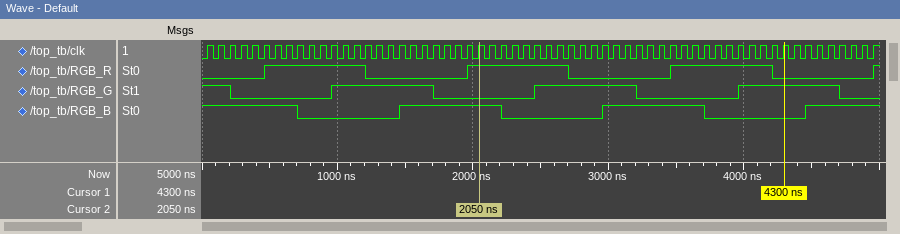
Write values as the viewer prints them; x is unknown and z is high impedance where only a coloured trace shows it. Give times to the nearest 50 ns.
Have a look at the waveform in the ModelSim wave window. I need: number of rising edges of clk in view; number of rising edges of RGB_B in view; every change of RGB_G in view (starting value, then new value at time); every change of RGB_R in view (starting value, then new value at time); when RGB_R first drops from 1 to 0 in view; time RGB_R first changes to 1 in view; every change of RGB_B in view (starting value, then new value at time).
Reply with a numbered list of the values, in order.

1. 60
2. 3
3. 1, 0 at 200 ns, 1 at 950 ns, 0 at 1700 ns, 1 at 2450 ns, 0 at 3200 ns, 1 at 3950 ns, 0 at 4700 ns
4. 0, 1 at 450 ns, 0 at 1200 ns, 1 at 1950 ns, 0 at 2700 ns, 1 at 3450 ns, 0 at 4200 ns, 1 at 4950 ns
5. 1200 ns
6. 450 ns
7. 1, 0 at 700 ns, 1 at 1450 ns, 0 at 2200 ns, 1 at 2950 ns, 0 at 3700 ns, 1 at 4450 ns
